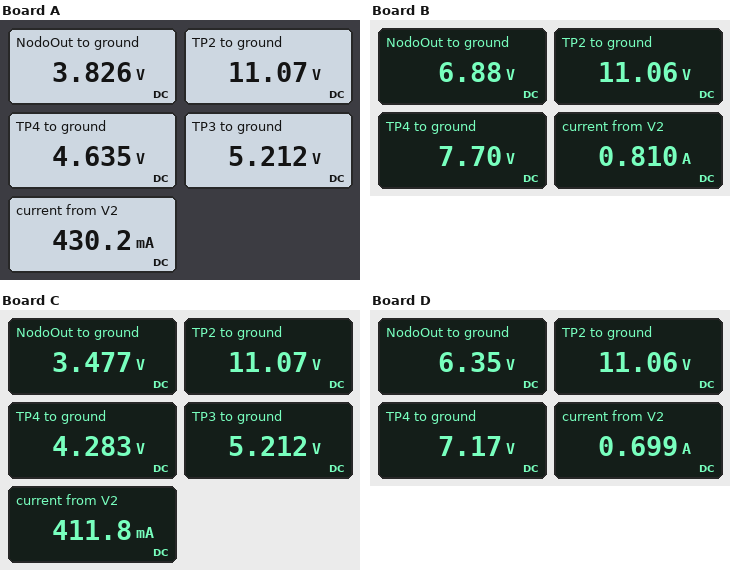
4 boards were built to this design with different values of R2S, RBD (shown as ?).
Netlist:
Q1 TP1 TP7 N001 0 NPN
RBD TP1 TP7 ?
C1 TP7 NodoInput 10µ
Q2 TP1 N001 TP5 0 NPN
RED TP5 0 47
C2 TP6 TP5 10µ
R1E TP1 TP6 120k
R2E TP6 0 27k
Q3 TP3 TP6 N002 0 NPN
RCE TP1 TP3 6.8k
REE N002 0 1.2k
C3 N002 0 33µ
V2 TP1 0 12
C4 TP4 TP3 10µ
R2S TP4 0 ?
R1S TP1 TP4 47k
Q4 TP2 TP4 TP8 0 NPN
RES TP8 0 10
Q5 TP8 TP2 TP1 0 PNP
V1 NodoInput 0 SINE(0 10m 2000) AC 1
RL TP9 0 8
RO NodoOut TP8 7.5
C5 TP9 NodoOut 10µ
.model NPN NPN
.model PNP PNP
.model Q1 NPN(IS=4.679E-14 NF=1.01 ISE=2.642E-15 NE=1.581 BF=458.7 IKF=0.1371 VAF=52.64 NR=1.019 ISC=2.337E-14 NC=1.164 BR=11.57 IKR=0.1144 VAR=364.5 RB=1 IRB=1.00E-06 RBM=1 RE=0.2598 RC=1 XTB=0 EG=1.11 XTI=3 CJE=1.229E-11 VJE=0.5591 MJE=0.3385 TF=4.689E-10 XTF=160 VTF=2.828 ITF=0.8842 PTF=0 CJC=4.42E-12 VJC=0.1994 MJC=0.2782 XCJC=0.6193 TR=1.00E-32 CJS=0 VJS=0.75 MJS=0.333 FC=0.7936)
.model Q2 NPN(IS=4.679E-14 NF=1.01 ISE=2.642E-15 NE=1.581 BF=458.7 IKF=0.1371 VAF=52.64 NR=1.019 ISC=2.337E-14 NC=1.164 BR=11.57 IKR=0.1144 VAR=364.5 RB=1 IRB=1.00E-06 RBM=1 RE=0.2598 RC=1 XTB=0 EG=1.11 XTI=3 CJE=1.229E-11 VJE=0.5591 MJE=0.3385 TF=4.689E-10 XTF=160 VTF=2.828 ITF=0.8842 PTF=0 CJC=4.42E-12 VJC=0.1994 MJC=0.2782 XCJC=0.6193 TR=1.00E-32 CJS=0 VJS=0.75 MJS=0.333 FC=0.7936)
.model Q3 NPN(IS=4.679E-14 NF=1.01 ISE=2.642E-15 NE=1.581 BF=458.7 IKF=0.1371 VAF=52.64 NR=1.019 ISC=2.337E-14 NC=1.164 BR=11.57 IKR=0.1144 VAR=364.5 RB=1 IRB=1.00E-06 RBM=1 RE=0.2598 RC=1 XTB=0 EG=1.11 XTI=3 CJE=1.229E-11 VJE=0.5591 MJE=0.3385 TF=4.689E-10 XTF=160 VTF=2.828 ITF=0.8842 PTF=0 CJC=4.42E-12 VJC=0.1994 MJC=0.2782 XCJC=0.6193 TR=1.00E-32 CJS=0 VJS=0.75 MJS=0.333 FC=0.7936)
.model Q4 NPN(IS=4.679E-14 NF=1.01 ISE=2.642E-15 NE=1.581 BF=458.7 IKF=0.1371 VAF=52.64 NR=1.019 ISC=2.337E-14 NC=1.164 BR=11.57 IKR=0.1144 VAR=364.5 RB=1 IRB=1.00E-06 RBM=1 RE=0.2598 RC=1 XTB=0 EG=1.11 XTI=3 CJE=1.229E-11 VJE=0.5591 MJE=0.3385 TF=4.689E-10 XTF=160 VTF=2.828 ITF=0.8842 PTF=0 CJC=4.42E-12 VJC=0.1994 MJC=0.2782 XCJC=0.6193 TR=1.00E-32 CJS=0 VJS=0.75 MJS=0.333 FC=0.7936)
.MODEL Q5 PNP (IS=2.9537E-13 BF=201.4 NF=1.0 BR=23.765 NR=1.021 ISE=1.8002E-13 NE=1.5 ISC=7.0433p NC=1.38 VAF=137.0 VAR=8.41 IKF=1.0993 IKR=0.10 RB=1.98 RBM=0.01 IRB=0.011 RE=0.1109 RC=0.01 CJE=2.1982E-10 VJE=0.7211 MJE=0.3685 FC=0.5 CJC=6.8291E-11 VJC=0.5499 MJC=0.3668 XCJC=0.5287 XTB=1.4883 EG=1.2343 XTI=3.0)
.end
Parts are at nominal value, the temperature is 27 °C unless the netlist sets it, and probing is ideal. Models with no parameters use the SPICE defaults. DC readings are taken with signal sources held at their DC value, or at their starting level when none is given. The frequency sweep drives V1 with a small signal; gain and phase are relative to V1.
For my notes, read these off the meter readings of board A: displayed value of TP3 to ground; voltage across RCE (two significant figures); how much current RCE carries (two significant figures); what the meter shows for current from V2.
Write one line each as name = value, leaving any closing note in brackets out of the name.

displayed value of TP3 to ground = 5.212 V
voltage across RCE = 6.8 V
how much current RCE carries = 1.0 mA
what the meter shows for current from V2 = 430.2 mA
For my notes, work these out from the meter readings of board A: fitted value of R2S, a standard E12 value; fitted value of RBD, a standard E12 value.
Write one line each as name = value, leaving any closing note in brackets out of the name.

fitted value of R2S, a standard E12 value = 39 kΩ
fitted value of RBD, a standard E12 value = 1.8 MΩ
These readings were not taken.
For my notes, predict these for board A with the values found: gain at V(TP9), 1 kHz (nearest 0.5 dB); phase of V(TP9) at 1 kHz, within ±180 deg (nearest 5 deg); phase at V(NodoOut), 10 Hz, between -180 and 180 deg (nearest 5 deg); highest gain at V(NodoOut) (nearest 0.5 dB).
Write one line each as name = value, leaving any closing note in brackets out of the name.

gain at V(TP9), 1 kHz = 36.0 dB
phase of V(TP9) at 1 kHz, within ±180 deg = -125 deg
phase at V(NodoOut), 10 Hz, between -180 and 180 deg = -105 deg
highest gain at V(NodoOut) = 44.0 dB
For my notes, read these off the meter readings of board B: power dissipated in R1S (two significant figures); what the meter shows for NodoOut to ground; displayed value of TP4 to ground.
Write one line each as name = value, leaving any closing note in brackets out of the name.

power dissipated in R1S = 390 µW
what the meter shows for NodoOut to ground = 6.88 V
displayed value of TP4 to ground = 7.70 V
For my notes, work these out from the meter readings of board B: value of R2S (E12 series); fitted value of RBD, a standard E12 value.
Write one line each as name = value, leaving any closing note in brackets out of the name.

value of R2S = 330 kΩ
fitted value of RBD, a standard E12 value = 390 kΩ
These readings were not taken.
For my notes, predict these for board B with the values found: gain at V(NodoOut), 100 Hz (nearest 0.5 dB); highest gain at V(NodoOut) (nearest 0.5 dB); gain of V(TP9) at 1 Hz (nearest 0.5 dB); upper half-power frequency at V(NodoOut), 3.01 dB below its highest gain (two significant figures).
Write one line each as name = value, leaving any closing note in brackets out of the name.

gain at V(NodoOut), 100 Hz = 39.5 dB
highest gain at V(NodoOut) = 45.0 dB
gain of V(TP9) at 1 Hz = -56.0 dB
upper half-power frequency at V(NodoOut), 3.01 dB below its highest gain = 2.3 kHz
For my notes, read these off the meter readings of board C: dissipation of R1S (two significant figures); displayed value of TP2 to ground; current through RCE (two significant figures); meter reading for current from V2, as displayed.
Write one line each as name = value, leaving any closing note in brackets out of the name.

dissipation of R1S = 1.3 mW
displayed value of TP2 to ground = 11.07 V
current through RCE = 1.0 mA
meter reading for current from V2, as displayed = 411.8 mA
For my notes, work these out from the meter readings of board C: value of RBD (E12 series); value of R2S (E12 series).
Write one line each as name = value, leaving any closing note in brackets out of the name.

value of RBD = 1.2 MΩ
value of R2S = 33 kΩ
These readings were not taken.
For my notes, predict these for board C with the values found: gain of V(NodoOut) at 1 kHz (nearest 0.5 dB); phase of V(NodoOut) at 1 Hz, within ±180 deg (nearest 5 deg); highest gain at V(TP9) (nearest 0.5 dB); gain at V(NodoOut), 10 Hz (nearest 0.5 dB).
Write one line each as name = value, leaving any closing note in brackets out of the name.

gain of V(NodoOut) at 1 kHz = 43.0 dB
phase of V(NodoOut) at 1 Hz, within ±180 deg = -90 deg
highest gain at V(TP9) = 39.0 dB
gain at V(NodoOut), 10 Hz = 20.0 dB
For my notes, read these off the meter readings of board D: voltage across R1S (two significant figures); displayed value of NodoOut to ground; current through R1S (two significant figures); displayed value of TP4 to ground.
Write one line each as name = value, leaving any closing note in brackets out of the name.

voltage across R1S = 4.8 V
displayed value of NodoOut to ground = 6.35 V
current through R1S = 100 µA
displayed value of TP4 to ground = 7.17 V
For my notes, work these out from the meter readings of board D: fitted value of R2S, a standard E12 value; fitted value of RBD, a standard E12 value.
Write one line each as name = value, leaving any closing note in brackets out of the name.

fitted value of R2S, a standard E12 value = 180 kΩ
fitted value of RBD, a standard E12 value = 1.2 MΩ
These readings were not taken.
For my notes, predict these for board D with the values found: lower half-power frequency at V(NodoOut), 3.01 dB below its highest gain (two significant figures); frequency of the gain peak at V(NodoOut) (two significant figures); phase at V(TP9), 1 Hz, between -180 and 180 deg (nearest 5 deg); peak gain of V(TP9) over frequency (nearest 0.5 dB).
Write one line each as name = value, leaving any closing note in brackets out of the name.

lower half-power frequency at V(NodoOut), 3.01 dB below its highest gain = 150 Hz
frequency of the gain peak at V(NodoOut) = 490 Hz
phase at V(TP9), 1 Hz, between -180 and 180 deg = -10 deg
peak gain of V(TP9) over frequency = 40.0 dB
